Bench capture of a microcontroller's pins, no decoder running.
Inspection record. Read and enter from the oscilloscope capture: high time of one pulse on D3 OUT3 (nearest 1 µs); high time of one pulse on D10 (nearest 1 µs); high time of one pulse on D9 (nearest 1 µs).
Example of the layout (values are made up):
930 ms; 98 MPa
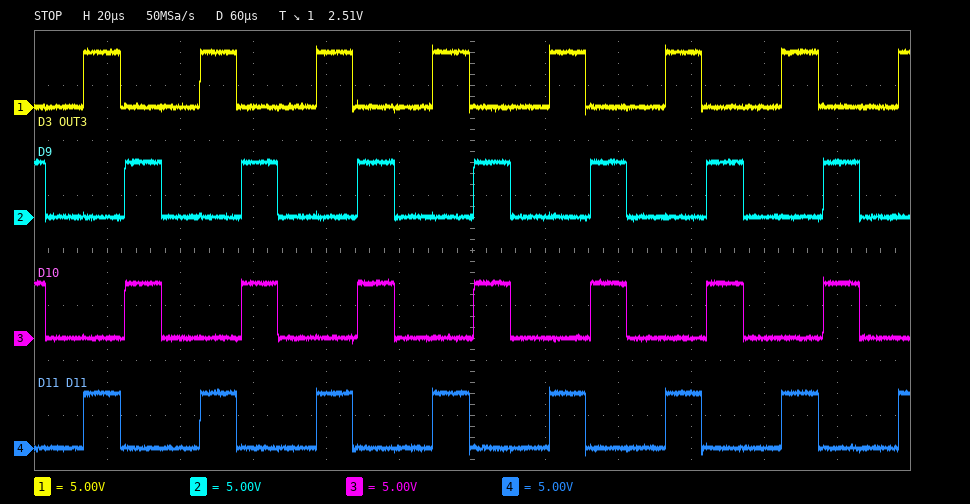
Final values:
10 µs; 10 µs; 10 µs
